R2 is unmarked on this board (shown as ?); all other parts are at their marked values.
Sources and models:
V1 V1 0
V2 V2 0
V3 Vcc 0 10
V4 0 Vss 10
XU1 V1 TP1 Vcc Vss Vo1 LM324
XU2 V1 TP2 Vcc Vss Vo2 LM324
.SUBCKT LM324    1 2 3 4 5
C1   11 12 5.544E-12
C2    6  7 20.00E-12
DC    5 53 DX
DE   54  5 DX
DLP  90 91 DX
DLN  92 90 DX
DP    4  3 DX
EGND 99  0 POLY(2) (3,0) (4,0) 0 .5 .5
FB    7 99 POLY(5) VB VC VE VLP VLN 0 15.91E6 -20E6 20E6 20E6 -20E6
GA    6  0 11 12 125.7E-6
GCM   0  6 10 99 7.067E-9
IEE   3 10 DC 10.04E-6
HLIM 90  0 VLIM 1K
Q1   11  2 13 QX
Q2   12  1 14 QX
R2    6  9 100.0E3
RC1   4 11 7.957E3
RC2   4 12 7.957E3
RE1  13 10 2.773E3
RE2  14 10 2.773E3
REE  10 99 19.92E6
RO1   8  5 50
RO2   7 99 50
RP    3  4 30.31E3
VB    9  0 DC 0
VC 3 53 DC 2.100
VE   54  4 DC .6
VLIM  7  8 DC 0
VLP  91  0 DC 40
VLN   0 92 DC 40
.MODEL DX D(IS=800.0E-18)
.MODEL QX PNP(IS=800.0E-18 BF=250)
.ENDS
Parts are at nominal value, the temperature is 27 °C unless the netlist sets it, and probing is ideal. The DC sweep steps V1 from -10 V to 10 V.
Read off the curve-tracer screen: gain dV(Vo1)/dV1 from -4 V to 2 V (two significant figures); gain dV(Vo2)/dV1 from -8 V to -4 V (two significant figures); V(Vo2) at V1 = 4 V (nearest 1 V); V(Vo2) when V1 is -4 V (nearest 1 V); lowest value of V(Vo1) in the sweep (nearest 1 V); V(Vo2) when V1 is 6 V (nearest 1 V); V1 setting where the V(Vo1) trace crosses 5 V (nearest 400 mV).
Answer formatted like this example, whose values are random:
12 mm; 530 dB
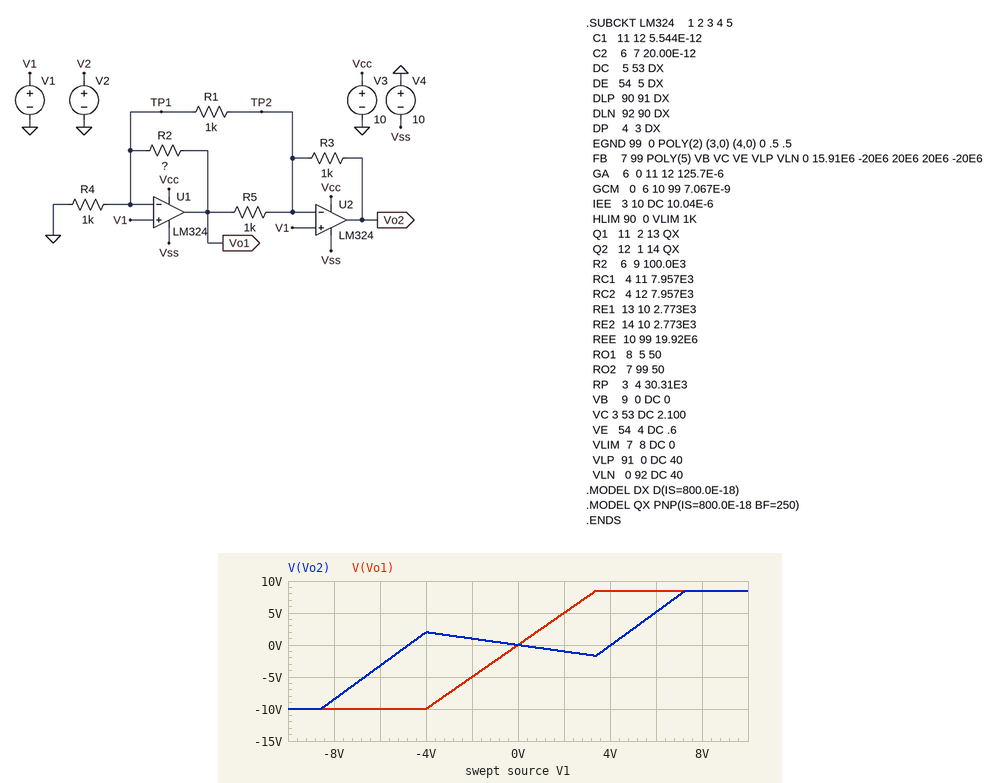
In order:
2.5 V/V; 2.6 V/V; 0 V; 2 V; -10 V; 5 V; 2.0 V
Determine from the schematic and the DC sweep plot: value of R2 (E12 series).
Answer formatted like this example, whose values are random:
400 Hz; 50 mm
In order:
1.5 kΩ
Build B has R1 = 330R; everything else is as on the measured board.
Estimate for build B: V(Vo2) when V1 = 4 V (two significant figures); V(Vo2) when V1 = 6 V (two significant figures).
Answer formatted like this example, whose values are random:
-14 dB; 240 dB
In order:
150 mV; 6.3 V
